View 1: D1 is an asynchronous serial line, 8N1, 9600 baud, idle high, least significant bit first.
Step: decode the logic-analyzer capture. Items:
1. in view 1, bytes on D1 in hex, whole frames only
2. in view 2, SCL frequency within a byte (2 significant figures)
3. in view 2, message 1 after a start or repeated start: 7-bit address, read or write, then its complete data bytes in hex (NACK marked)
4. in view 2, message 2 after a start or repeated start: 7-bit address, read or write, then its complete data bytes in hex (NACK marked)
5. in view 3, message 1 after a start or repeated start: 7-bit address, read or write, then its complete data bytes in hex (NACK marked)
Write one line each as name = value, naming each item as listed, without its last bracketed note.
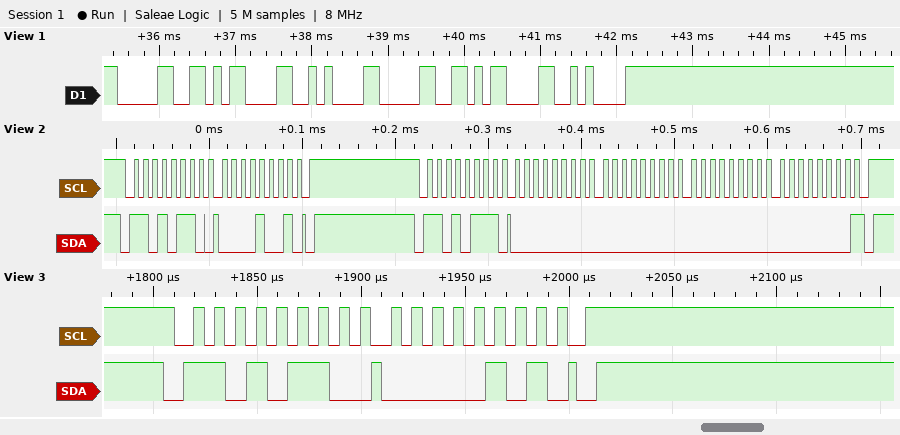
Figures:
in view 1, bytes on D1 in hex, whole frames only = 30 0D 0A 30 0D 0A
in view 2, SCL frequency within a byte = 100 kHz
in view 2, message 1 after a start or repeated start: 7-bit address, read or write, then its complete data bytes in hex = 0x6B write: 09
in view 2, message 2 after a start or repeated start: 7-bit address, read or write, then its complete data bytes in hex = 0x6B read: 00 00 00 00 NACK
in view 3, message 1 after a start or repeated start: 7-bit address, read or write, then its complete data bytes in hex = 0x6B write: 05
